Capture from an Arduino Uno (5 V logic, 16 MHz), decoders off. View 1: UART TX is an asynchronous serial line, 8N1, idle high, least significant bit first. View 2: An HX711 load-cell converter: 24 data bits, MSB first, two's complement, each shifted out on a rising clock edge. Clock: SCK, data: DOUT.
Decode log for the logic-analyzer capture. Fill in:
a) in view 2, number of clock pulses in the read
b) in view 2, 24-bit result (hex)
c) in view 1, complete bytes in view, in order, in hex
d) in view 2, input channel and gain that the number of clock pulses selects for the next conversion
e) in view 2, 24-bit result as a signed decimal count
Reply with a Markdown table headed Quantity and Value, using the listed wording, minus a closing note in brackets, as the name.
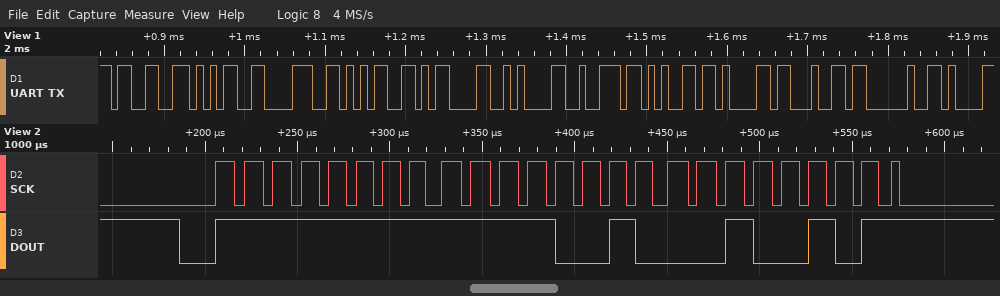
| Quantity | Value |
|---|---|
| in view 2, number of clock pulses in the read | 25 |
| in view 2, 24-bit result | 0xFFF225 |
| in view 1, complete bytes in view, in order, in hex | 0x33 0x35 0x38 0x35 0x0D 0x0A 0x72 0x65 0x61 0x64 0x20 |
| in view 2, input channel and gain that the number of clock pulses selects for the next conversion | channel A, gain 128 |
| in view 2, 24-bit result as a signed decimal count | -3547 |
